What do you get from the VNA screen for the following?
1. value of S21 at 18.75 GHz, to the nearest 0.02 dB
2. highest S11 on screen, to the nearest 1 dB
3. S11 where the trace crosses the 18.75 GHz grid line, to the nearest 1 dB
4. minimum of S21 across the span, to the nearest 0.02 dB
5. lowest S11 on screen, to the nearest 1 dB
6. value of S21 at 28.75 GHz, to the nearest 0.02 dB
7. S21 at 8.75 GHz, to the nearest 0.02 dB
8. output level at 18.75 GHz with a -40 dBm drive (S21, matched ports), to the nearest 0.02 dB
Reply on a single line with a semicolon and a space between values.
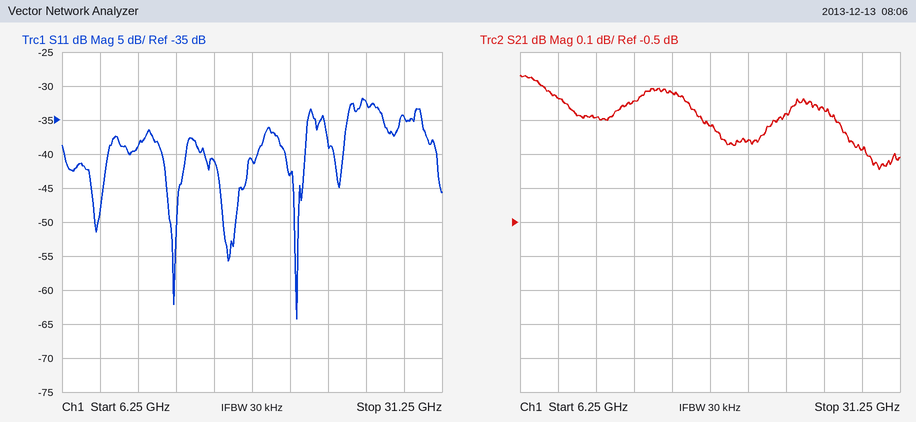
-0.22 dB; -32 dB; -41 dB; -0.34 dB; -64 dB; -0.28 dB; -0.14 dB; -40.22 dBm
